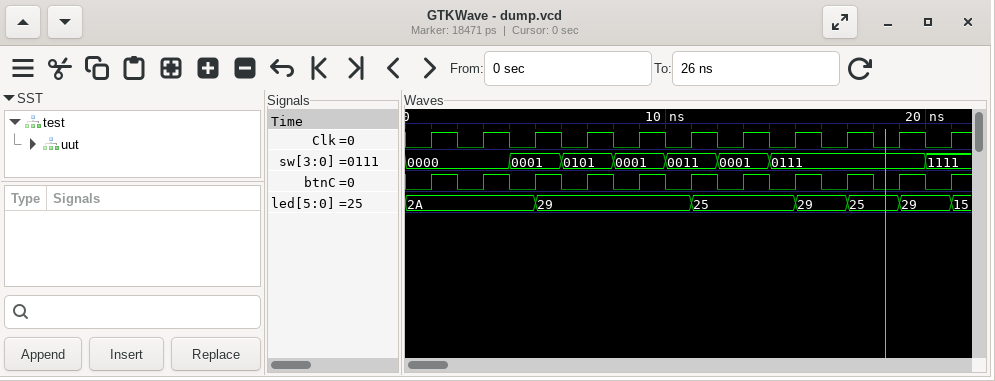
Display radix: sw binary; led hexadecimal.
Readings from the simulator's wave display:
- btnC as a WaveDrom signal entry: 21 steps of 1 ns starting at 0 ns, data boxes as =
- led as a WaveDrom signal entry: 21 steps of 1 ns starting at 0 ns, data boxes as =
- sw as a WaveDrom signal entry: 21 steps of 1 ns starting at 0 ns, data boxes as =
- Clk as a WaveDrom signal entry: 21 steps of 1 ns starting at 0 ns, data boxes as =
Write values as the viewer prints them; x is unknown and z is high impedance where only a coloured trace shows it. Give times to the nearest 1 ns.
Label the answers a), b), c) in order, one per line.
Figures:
a) {name: 'btnC', wave: '010101010101010101010'}
b) {name: 'led', wave: '=....=.....=...=.=.=.', data: '2A 29 25 29 25 29'}
c) {name: 'sw', wave: '=...=.=.=.=.=.=.....=', data: '0000 0001 0101 0001 0011 0001 0111 1111'}
d) {name: 'Clk', wave: '010101010101010101010'}
